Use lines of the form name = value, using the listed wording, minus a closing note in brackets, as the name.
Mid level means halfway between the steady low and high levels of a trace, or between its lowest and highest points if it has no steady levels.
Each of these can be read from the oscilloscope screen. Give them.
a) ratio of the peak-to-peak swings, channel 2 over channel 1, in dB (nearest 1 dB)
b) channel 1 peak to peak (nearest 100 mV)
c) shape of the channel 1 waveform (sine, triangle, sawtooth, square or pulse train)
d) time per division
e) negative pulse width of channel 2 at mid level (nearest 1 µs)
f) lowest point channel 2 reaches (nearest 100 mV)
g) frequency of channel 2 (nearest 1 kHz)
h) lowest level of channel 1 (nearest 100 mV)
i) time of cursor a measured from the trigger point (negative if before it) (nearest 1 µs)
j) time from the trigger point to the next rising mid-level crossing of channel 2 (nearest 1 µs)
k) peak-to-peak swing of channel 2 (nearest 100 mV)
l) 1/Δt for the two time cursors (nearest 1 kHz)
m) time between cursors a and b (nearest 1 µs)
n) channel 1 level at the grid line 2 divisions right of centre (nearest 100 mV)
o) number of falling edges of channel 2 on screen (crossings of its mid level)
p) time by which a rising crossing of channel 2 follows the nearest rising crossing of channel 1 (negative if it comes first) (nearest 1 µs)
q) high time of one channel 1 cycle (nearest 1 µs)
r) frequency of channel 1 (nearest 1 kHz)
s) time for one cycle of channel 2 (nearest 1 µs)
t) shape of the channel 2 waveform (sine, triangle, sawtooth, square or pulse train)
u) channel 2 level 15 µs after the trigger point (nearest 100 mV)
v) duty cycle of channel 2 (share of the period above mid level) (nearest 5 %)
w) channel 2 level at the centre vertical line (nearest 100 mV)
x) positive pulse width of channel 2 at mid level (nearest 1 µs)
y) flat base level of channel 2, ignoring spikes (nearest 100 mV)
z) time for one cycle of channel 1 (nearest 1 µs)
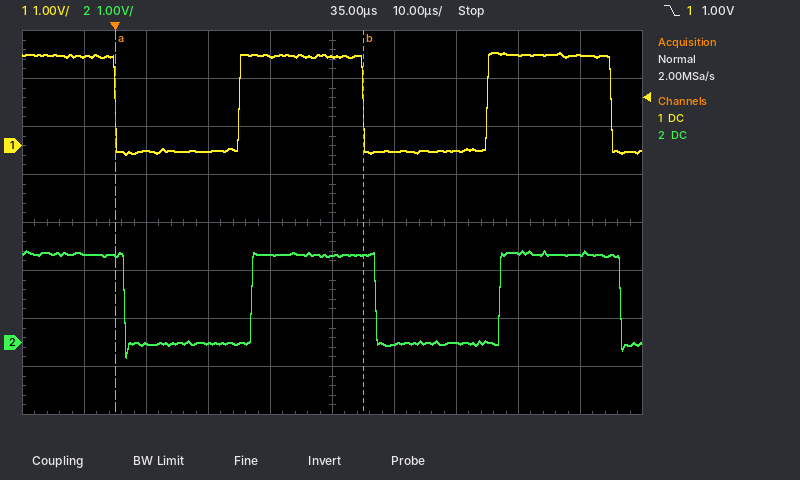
ratio of the peak-to-peak swings, channel 2 over channel 1, in dB = 0 dB
channel 1 peak to peak = 2.1 V
shape of the channel 1 waveform = square
time per division = 10 µs
negative pulse width of channel 2 at mid level = 20 µs
lowest point channel 2 reaches = -300 mV
frequency of channel 2 = 25 kHz
lowest level of channel 1 = -200 mV
time of cursor a measured from the trigger point (negative if before it) = 0 µs
time from the trigger point to the next rising mid-level crossing of channel 2 = 22 µs
peak-to-peak swing of channel 2 = 2.2 V
1/Δt for the two time cursors = 25 kHz
time between cursors a and b = 40 µs
channel 1 level at the grid line 2 divisions right of centre = -100 mV
number of falling edges of channel 2 on screen = 3
time by which a rising crossing of channel 2 follows the nearest rising crossing of channel 1 (negative if it comes first) = +2 µs
high time of one channel 1 cycle = 20 µs
frequency of channel 1 = 25 kHz
time for one cycle of channel 2 = 40 µs
shape of the channel 2 waveform = square
channel 2 level 15 µs after the trigger point = 0.0 V
duty cycle of channel 2 (share of the period above mid level) = 50 %
channel 2 level at the centre vertical line = 1.8 V
positive pulse width of channel 2 at mid level = 20 µs
flat base level of channel 2, ignoring spikes = 0.0 V
time for one cycle of channel 1 = 40 µs
